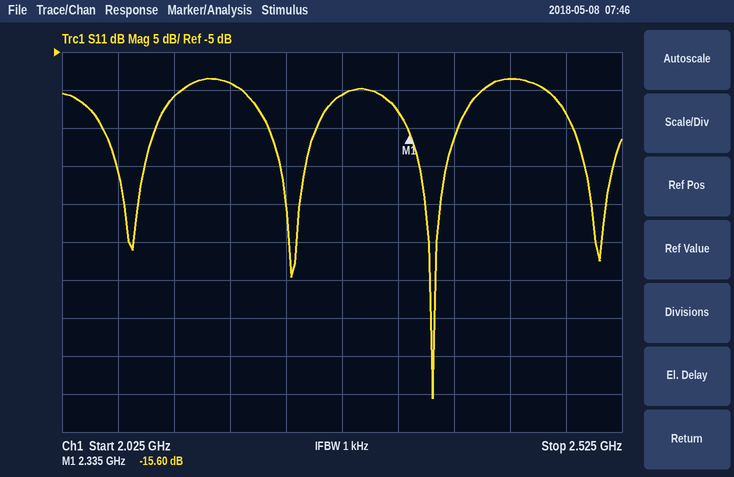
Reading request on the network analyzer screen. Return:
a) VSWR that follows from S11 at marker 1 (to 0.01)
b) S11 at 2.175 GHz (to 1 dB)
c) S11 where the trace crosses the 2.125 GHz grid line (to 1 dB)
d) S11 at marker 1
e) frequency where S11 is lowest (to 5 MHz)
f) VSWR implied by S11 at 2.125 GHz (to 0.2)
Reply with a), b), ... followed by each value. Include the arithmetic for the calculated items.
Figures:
a) (1 + 0.1660)/(1 − 0.1660) ≈ 1.40
b) -9 dB
c) -11 dB
d) -15.60 dB
e) 2.355 GHz
f) |Γ| = 10^(-11/20) = 0.2818; VSWR = (1 + 0.2818)/(1 − 0.2818) ≈ 1.8
